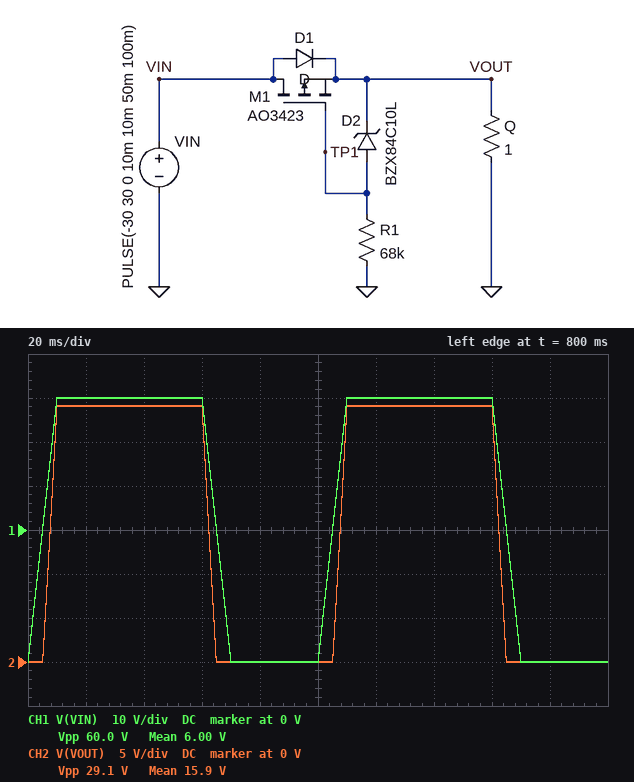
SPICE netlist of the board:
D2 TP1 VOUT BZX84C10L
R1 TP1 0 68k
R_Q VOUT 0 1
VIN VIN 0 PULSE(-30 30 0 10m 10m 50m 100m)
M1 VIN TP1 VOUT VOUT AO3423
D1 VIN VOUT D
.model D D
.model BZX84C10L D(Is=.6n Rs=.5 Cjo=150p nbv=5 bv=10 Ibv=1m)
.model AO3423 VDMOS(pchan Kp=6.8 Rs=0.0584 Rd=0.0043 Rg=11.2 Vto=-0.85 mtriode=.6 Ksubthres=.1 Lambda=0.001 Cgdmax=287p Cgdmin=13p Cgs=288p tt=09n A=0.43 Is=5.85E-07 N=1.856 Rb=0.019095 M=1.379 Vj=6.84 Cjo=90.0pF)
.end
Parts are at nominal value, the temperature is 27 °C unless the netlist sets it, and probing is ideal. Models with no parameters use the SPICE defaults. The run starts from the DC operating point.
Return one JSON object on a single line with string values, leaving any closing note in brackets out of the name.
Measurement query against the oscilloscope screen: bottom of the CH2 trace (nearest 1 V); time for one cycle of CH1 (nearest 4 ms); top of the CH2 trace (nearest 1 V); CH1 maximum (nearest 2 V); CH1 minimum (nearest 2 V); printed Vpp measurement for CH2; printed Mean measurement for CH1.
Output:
{"bottom of the CH2 trace": "0 V", "time for one cycle of CH1": "100 ms", "top of the CH2 trace": "29 V", "CH1 maximum": "30 V", "CH1 minimum": "-30 V", "printed Vpp measurement for CH2": "29.1 V", "printed Mean measurement for CH1": "6.00 V"}
